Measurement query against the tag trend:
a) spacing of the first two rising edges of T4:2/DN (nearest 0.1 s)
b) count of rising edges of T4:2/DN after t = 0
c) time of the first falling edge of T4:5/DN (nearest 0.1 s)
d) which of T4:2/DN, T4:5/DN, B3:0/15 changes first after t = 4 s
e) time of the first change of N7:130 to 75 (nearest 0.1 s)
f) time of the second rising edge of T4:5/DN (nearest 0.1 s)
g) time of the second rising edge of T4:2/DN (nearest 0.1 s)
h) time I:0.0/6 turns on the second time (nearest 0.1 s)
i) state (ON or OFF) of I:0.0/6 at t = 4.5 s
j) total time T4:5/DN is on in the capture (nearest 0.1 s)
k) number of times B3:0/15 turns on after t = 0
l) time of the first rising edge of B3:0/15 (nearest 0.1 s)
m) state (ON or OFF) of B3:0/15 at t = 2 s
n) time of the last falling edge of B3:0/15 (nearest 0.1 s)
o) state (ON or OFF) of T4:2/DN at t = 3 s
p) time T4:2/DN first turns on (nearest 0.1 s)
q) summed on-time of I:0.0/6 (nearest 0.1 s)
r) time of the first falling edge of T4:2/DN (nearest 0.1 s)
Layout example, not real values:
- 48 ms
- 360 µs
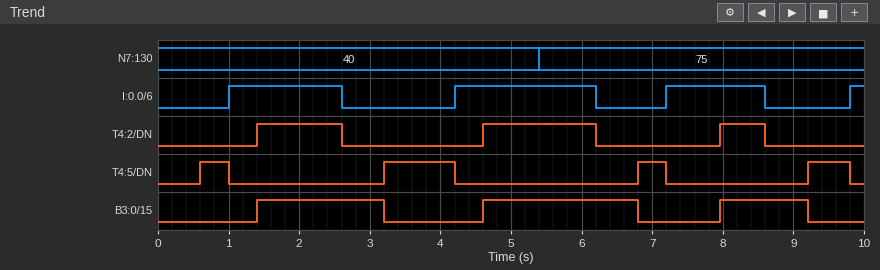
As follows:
- 3.2 s
- 3
- 1.0 s
- T4:5/DN
- 5.4 s
- 3.2 s
- 4.6 s
- 4.2 s
- ON
- 2.4 s
- 3
- 1.4 s
- ON
- 9.2 s
- OFF
- 1.4 s
- 5.2 s
- 2.6 s
